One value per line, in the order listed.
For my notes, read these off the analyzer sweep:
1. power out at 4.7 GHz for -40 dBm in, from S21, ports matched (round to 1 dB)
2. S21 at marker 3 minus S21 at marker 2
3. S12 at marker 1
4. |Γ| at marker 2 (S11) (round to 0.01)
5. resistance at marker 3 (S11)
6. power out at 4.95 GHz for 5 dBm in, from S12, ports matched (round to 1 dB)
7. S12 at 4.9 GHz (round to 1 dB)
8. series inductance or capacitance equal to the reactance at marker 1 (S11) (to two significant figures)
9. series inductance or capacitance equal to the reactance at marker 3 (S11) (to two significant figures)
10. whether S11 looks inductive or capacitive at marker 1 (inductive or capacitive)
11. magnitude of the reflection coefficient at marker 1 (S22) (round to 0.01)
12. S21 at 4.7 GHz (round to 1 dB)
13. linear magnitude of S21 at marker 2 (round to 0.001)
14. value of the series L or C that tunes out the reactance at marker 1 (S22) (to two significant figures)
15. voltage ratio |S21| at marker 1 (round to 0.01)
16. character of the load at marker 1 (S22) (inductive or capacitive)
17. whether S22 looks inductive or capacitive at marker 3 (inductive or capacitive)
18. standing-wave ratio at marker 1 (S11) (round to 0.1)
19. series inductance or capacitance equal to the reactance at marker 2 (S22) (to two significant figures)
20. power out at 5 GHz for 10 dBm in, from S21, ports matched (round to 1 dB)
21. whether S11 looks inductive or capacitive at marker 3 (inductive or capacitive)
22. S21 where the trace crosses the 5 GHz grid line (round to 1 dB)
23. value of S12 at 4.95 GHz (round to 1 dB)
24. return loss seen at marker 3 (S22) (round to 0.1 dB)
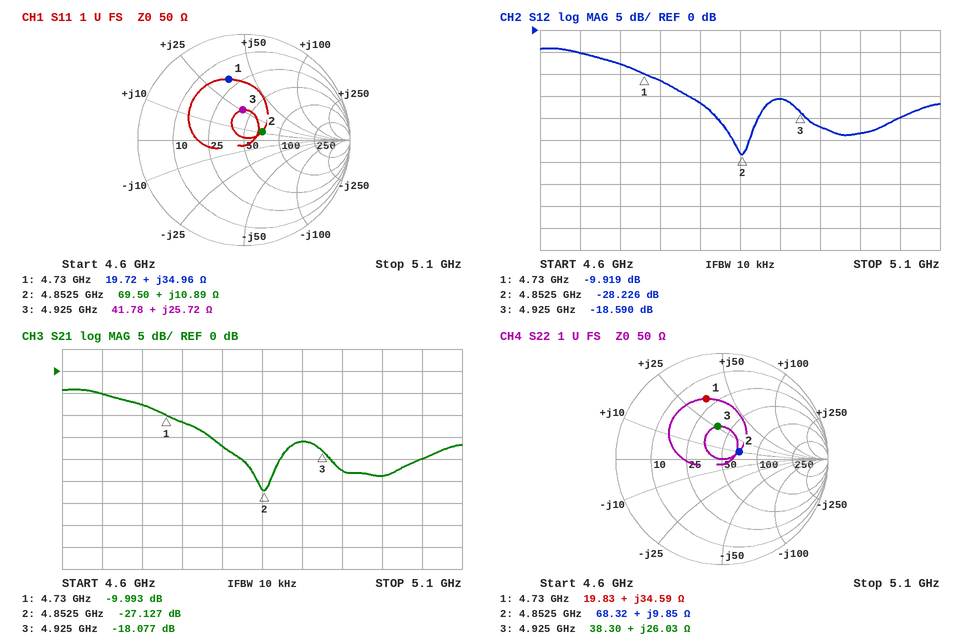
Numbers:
-48 dBm
9.050 dB
-9.919 dB
0.19
41.78 Ω
-17 dBm
-16 dB
1.2 nH
830 pH
inductive
0.59
-8 dB
0.044
970 fF
0.32
inductive
inductive
3.9
320 pH
-14 dBm
inductive
-24 dB
-22 dB
10.2 dB
